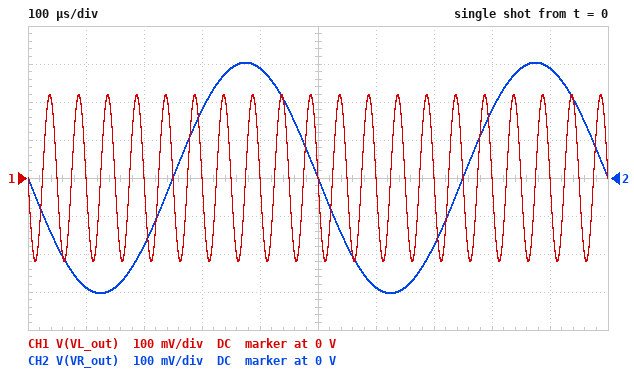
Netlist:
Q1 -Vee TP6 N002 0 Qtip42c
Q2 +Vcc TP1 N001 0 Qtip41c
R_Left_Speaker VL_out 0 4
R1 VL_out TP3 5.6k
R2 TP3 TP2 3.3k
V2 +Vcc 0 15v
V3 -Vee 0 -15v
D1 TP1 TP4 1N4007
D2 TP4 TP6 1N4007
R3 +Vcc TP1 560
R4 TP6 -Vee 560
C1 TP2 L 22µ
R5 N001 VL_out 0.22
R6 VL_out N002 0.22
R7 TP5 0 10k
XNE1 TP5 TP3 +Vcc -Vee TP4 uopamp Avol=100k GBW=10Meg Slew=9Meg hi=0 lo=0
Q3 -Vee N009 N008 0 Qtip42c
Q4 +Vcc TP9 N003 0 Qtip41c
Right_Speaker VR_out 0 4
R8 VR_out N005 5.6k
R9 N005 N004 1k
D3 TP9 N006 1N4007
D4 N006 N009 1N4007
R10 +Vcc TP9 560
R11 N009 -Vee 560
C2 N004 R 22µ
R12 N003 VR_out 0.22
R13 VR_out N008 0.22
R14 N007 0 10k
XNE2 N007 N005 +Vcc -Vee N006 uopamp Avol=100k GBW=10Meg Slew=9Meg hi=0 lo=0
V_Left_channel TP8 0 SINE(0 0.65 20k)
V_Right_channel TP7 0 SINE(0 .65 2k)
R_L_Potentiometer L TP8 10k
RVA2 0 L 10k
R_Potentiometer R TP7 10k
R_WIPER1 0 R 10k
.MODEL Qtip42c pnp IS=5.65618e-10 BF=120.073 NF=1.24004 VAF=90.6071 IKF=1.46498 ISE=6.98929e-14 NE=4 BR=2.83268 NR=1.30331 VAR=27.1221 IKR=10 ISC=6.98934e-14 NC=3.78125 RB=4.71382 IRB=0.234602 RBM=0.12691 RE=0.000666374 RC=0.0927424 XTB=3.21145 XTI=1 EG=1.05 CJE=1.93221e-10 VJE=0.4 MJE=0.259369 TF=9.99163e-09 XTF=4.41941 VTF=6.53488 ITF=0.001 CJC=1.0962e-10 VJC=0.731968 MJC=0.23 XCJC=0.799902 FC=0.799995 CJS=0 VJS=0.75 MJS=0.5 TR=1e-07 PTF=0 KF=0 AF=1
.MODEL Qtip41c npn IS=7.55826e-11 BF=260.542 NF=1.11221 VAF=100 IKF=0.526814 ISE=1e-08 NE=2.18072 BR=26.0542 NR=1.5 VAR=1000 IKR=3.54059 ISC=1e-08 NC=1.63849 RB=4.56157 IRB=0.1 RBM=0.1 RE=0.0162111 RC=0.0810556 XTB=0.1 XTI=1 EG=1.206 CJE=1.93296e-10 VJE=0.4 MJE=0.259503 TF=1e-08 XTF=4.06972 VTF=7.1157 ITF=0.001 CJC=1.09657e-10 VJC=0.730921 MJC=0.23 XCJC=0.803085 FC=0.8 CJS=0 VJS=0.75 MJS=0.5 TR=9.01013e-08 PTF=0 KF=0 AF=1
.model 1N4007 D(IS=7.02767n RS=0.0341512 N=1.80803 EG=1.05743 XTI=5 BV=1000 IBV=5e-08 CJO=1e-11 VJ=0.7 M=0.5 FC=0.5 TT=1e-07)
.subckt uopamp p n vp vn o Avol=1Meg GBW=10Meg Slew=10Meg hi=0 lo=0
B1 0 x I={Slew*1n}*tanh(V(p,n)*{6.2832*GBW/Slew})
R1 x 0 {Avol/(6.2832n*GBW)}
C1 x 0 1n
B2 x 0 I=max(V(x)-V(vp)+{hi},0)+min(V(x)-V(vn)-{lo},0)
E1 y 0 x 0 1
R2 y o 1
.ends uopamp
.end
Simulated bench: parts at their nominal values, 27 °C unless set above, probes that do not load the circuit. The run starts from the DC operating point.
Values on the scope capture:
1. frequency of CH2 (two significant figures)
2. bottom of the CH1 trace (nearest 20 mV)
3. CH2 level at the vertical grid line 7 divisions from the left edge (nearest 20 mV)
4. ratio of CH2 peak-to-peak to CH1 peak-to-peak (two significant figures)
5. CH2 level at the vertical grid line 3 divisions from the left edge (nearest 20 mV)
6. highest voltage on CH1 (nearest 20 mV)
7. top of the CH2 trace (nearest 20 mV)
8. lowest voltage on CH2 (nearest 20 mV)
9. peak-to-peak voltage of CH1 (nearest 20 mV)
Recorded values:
2.0 kHz
-220 mV
-180 mV
1.4
180 mV
220 mV
300 mV
-300 mV
440 mV
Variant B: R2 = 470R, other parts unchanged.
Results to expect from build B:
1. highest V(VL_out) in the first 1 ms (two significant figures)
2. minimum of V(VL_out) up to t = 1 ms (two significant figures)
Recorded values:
330 mV
-330 mV
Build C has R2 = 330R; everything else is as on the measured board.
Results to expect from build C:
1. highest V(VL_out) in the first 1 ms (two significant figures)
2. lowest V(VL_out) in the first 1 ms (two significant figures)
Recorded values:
340 mV
-340 mV
